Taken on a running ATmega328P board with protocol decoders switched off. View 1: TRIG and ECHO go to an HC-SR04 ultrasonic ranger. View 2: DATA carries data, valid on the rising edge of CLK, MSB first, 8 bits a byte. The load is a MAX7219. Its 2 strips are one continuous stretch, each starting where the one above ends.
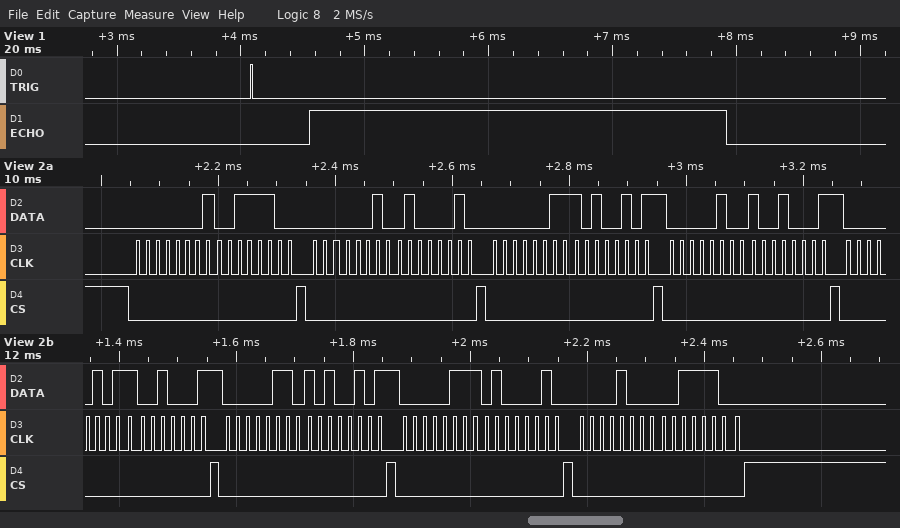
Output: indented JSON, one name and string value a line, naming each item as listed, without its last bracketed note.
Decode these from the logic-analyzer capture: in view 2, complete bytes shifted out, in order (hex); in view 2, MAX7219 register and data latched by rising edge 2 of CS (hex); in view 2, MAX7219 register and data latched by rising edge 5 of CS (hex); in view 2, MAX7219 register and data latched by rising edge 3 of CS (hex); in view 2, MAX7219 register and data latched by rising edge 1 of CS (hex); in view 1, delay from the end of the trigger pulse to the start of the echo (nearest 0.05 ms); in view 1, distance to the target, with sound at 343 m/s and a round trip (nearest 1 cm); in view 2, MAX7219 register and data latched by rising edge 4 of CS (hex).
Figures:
{
  "in view 2, complete bytes shifted out, in order": "01 3C 02 42 03 A5 04 91 05 91 06 A5 07 42 08 3C",
  "in view 2, MAX7219 register and data latched by rising edge 2 of CS": "register 0x2, data 0x42",
  "in view 2, MAX7219 register and data latched by rising edge 5 of CS": "register 0x5, data 0x91",
  "in view 2, MAX7219 register and data latched by rising edge 3 of CS": "register 0x3, data 0xA5",
  "in view 2, MAX7219 register and data latched by rising edge 1 of CS": "register 0x1, data 0x3C",
  "in view 1, delay from the end of the trigger pulse to the start of the echo": "0.45 ms",
  "in view 1, distance to the target, with sound at 343 m/s and a round trip": "58 cm",
  "in view 2, MAX7219 register and data latched by rising edge 4 of CS": "register 0x4, data 0x91"
}
